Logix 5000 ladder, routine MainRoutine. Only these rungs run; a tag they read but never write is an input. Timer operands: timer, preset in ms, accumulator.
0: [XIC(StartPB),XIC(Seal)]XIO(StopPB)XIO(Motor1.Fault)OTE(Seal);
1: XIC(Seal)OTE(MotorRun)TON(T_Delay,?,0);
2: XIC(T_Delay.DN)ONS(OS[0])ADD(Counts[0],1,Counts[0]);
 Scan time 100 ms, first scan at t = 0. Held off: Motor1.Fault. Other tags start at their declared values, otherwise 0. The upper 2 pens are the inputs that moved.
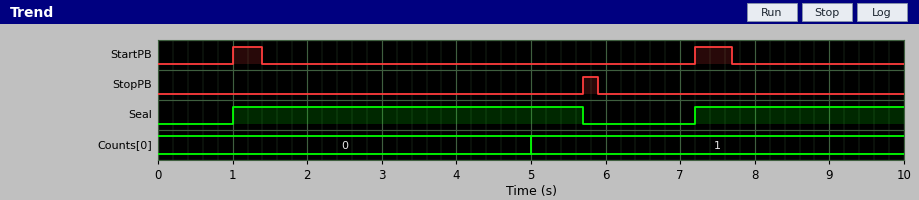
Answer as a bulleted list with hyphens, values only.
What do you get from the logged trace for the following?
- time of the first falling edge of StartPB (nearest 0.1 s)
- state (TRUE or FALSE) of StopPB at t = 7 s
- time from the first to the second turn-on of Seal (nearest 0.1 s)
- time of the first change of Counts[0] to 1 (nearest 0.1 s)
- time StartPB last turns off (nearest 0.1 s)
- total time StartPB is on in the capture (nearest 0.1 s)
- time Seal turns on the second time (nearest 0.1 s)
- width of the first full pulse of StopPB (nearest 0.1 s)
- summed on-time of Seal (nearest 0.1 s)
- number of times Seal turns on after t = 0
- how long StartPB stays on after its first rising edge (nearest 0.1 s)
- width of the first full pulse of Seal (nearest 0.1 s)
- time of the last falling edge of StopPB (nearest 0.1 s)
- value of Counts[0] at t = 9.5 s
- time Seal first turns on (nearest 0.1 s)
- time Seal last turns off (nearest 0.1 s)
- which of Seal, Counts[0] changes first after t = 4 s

- 1.4 s
- FALSE
- 6.2 s
- 5.0 s
- 7.7 s
- 0.9 s
- 7.2 s
- 0.2 s
- 7.5 s
- 2
- 0.4 s
- 4.7 s
- 5.9 s
- 1
- 1.0 s
- 5.7 s
- Counts[0]
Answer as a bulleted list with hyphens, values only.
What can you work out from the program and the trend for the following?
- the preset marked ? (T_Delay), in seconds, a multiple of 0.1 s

- 4.0 s
